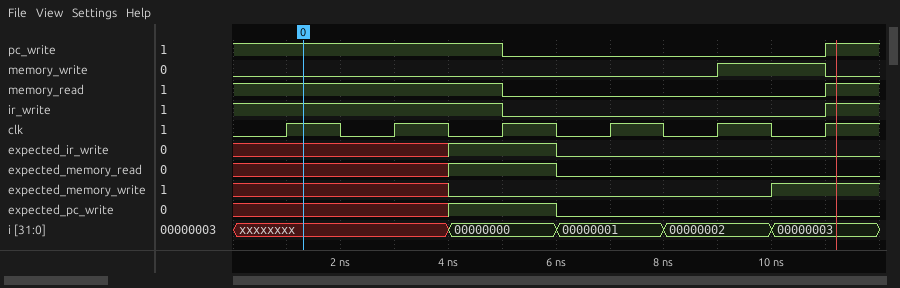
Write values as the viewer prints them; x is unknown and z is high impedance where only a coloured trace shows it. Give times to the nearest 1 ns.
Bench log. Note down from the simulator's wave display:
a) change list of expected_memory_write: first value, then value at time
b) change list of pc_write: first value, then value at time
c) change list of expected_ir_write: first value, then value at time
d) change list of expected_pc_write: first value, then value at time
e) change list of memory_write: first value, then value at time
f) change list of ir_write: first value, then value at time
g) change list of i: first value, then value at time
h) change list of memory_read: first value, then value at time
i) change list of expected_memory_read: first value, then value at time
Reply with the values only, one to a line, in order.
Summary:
x, 0 at 4 ns, 1 at 10 ns
1, 0 at 5 ns, 1 at 11 ns
x, 1 at 4 ns, 0 at 6 ns
x, 1 at 4 ns, 0 at 6 ns
0, 1 at 9 ns, 0 at 11 ns
1, 0 at 5 ns, 1 at 11 ns
xxxxxxxx, 00000000 at 4 ns, 00000001 at 6 ns, 00000002 at 8 ns, 00000003 at 10 ns
1, 0 at 5 ns, 1 at 11 ns
x, 1 at 4 ns, 0 at 6 ns
